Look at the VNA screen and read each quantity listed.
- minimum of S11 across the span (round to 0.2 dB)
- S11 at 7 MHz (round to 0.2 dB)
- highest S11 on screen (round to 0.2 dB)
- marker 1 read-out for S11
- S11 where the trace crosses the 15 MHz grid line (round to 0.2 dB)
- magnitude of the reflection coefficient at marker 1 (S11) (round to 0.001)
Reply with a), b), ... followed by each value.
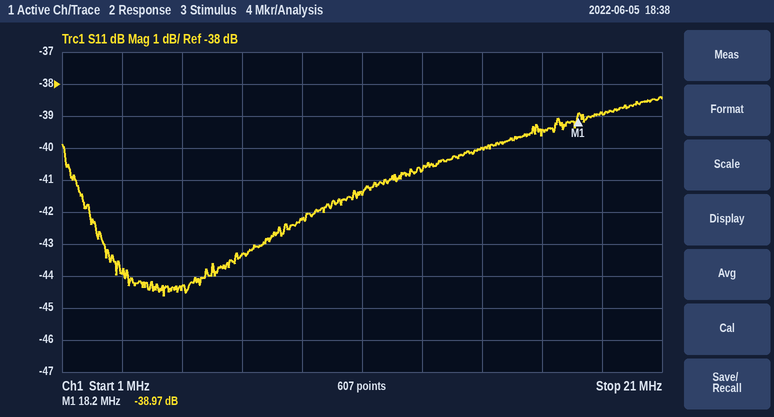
a) -44.6 dB
b) -43.4 dB
c) -38.4 dB
d) -38.97 dB
e) -40.0 dB
f) 0.011
